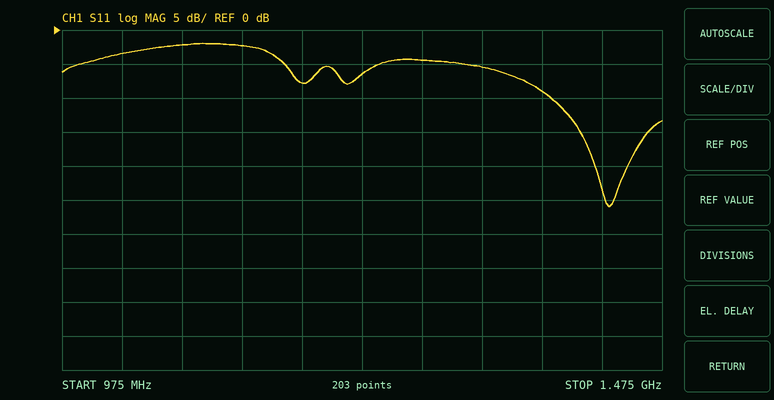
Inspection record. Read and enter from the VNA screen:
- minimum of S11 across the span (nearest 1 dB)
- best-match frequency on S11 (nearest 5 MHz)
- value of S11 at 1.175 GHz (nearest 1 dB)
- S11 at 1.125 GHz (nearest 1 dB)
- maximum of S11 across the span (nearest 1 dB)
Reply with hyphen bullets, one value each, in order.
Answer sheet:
- -26 dB
- 1.430 GHz
- -8 dB
- -2 dB
- -2 dB
